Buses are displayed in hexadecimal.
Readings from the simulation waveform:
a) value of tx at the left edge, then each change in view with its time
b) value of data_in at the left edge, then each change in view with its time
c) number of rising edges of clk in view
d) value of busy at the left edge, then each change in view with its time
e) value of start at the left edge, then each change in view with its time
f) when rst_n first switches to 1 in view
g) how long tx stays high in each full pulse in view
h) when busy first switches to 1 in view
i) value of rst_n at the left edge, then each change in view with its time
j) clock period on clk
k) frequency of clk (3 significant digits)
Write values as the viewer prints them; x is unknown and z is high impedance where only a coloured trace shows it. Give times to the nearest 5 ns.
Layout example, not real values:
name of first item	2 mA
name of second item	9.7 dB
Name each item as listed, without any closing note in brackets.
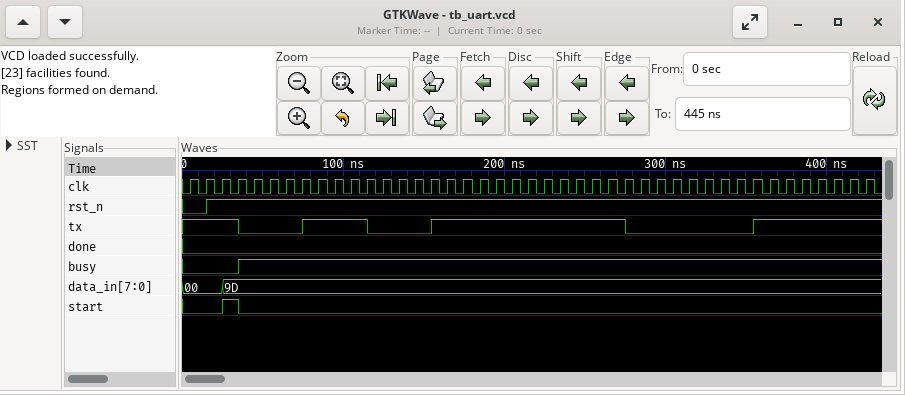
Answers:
value of tx at the left edge, then each change in view with its time	1, 0 at 35 ns, 1 at 75 ns, 0 at 115 ns, 1 at 155 ns, 0 at 275 ns, 1 at 355 ns
value of data_in at the left edge, then each change in view with its time	00, 9D at 25 ns
number of rising edges of clk in view	43
value of busy at the left edge, then each change in view with its time	0, 1 at 35 ns
value of start at the left edge, then each change in view with its time	0, 1 at 25 ns, 0 at 35 ns
when rst_n first switches to 1 in view	15 ns
how long tx stays high in each full pulse in view	40 ns, 120 ns
when busy first switches to 1 in view	35 ns
value of rst_n at the left edge, then each change in view with its time	0, 1 at 15 ns
clock period on clk	10 ns
frequency of clk	100 MHz
